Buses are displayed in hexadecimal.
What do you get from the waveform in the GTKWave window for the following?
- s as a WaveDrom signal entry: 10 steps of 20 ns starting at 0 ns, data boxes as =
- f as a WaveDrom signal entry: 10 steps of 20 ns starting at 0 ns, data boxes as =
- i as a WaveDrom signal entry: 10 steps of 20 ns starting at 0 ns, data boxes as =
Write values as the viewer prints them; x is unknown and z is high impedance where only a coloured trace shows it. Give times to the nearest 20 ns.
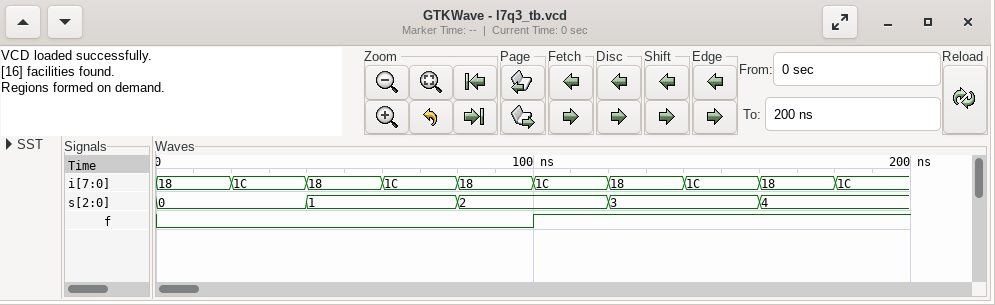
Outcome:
{name: 's', wave: '=.=.=.=.=.', data: '0 1 2 3 4'}
{name: 'f', wave: '0....1....'}
{name: 'i', wave: '==========', data: '18 1C 18 1C 18 1C 18 1C 18 1C'}
